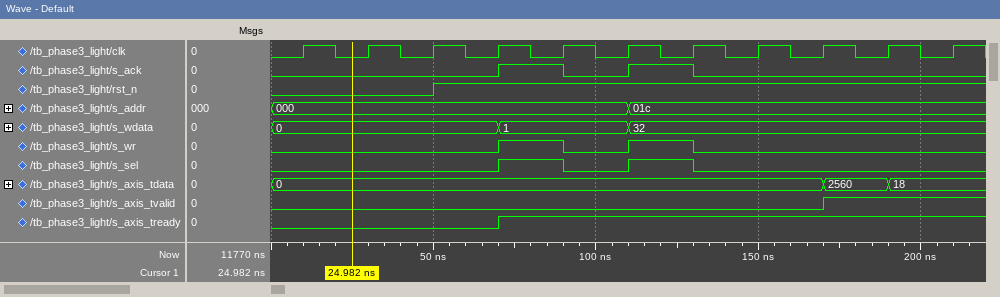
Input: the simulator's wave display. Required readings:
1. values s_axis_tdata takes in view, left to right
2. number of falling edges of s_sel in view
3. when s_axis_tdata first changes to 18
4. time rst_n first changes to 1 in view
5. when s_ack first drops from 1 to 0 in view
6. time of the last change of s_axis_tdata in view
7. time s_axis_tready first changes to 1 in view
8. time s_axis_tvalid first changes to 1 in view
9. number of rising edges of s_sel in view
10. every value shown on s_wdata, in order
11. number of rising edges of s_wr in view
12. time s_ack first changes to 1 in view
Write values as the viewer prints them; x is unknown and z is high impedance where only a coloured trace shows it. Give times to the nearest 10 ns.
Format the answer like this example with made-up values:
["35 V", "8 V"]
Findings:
["0, 2560, 18", "2", "190 ns", "50 ns", "90 ns", "190 ns", "70 ns", "170 ns", "2", "0, 1, 32", "2", "70 ns"]
